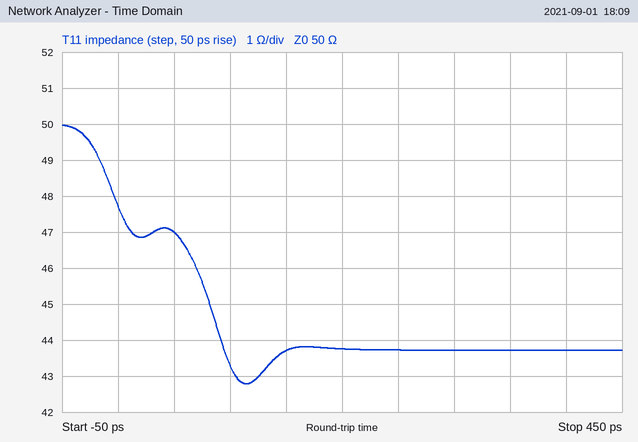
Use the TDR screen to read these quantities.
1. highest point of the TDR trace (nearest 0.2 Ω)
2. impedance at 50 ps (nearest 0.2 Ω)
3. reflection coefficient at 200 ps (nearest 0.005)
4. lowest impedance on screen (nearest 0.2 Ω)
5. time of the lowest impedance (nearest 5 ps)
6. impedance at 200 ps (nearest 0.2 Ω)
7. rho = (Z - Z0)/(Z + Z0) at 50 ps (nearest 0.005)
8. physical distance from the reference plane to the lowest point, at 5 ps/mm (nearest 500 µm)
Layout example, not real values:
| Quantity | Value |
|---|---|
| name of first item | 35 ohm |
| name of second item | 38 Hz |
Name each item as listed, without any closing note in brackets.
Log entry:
| Quantity | Value |
|---|---|
| highest point of the TDR trace | 50.0 Ω |
| impedance at 50 ps | 47.0 Ω |
| reflection coefficient at 200 ps | -0.065 |
| lowest impedance on screen | 42.8 Ω |
| time of the lowest impedance | 115 ps |
| impedance at 200 ps | 43.8 Ω |
| rho = (Z - Z0)/(Z + Z0) at 50 ps | -0.030 |
| physical distance from the reference plane to the lowest point, at 5 ps/mm | 11.5 mm |
